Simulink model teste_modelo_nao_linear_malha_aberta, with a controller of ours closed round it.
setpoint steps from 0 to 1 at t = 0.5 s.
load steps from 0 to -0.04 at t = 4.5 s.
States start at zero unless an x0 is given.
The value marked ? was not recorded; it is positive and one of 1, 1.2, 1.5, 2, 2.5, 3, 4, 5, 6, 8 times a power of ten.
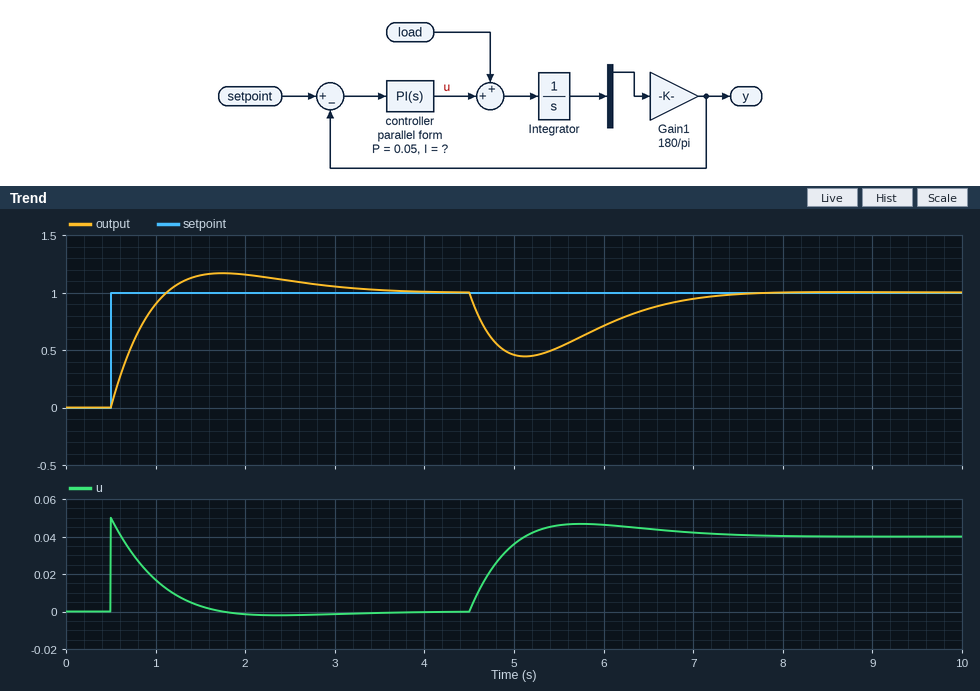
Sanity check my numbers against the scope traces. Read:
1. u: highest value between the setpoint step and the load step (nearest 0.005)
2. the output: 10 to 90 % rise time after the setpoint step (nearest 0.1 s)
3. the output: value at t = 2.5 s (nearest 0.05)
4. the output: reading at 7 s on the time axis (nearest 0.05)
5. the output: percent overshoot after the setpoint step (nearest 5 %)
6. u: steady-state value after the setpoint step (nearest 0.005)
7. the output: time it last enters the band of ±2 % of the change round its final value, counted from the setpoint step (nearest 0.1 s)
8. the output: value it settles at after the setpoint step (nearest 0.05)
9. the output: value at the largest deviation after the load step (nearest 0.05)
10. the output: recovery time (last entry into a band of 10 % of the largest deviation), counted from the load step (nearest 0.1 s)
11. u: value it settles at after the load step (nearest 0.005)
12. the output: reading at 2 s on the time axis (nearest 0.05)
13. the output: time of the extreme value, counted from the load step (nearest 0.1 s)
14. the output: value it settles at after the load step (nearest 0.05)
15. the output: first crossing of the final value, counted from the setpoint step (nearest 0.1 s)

0.050
0.5 s
1.10
0.95
15 %
0.000
3.0 s
1.00
0.45
2.5 s
0.040
1.15
0.6 s
1.00
0.6 s
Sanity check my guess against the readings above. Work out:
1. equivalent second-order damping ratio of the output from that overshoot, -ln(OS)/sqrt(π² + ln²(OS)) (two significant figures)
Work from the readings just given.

0.52
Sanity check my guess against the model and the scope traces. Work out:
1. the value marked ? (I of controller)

0.05
